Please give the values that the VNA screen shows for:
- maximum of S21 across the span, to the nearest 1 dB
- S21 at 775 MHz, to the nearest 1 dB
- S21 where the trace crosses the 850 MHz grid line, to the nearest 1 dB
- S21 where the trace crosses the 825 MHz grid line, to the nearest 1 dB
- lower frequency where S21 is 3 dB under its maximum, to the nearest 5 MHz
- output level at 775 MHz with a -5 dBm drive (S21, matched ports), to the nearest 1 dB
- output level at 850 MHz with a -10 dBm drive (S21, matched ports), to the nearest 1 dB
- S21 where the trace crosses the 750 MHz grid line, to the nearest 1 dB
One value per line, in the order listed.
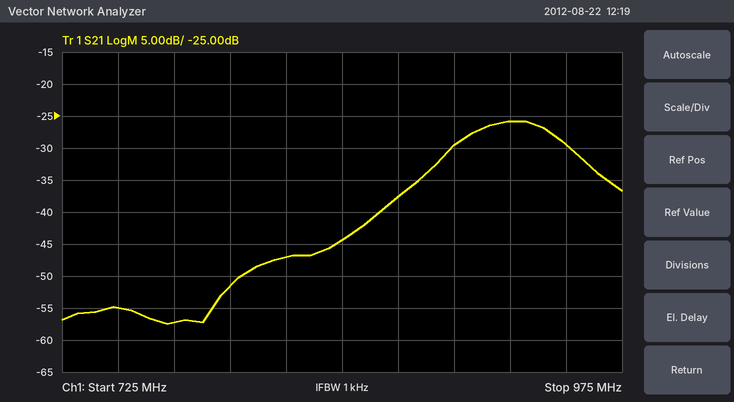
-26 dB
-57 dB
-44 dB
-47 dB
905 MHz
-62 dBm
-54 dBm
-55 dB
